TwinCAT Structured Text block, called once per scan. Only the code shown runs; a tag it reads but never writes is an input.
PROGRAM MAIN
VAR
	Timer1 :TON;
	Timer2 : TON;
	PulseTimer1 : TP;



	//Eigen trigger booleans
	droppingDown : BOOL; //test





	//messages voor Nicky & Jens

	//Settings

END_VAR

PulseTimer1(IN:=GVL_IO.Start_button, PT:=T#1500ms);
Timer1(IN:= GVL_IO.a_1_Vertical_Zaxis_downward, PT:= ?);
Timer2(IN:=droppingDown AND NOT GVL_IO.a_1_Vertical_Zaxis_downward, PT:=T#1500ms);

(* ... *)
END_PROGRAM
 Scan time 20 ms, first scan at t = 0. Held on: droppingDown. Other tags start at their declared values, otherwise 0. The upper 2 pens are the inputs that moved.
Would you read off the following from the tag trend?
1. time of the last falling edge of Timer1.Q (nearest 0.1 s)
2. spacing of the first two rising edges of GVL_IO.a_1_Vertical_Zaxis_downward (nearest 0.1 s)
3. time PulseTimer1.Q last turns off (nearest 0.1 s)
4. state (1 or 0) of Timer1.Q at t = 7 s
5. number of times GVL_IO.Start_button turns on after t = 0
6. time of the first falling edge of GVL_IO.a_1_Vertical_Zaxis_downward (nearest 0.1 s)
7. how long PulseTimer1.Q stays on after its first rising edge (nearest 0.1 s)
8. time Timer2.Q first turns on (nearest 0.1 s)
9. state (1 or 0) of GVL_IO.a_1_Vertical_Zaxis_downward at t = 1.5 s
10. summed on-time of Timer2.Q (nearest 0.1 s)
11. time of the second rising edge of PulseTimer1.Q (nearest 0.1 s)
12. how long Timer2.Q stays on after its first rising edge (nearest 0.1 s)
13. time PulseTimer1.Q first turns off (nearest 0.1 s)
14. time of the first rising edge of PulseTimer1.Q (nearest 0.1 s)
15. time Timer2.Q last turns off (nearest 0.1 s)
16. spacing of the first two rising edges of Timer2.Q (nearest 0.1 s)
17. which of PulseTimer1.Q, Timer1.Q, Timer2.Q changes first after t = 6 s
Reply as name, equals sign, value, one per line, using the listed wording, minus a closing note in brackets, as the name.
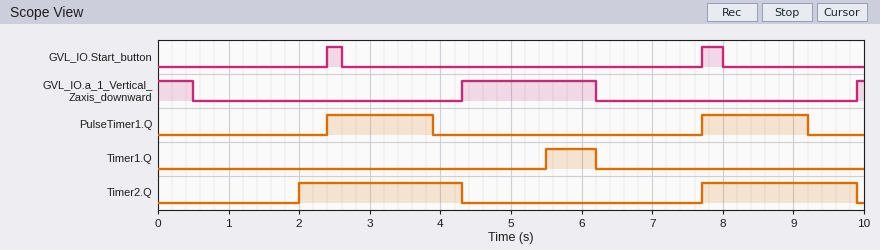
time of the last falling edge of Timer1.Q = 6.2 s
spacing of the first two rising edges of GVL_IO.a_1_Vertical_Zaxis_downward = 5.6 s
time PulseTimer1.Q last turns off = 9.2 s
state (1 or 0) of Timer1.Q at t = 7 s = 0
number of times GVL_IO.Start_button turns on after t = 0 = 2
time of the first falling edge of GVL_IO.a_1_Vertical_Zaxis_downward = 0.5 s
how long PulseTimer1.Q stays on after its first rising edge = 1.5 s
time Timer2.Q first turns on = 2.0 s
state (1 or 0) of GVL_IO.a_1_Vertical_Zaxis_downward at t = 1.5 s = 0
summed on-time of Timer2.Q = 4.5 s
time of the second rising edge of PulseTimer1.Q = 7.7 s
how long Timer2.Q stays on after its first rising edge = 2.3 s
time PulseTimer1.Q first turns off = 3.9 s
time of the first rising edge of PulseTimer1.Q = 2.4 s
time Timer2.Q last turns off = 9.9 s
spacing of the first two rising edges of Timer2.Q = 5.7 s
which of PulseTimer1.Q, Timer1.Q, Timer2.Q changes first after t = 6 s = Timer1.Q
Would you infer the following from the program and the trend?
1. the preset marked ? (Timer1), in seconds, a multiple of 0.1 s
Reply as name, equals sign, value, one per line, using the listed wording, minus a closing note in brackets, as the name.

the preset marked ? (Timer1), in seconds, a multiple of 0.1 s = 1.2 s
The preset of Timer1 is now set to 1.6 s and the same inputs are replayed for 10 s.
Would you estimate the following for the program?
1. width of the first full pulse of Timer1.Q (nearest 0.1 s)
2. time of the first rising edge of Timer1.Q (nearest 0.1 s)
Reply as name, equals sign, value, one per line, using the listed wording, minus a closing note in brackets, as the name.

width of the first full pulse of Timer1.Q = 0.3 s
time of the first rising edge of Timer1.Q = 5.9 s
